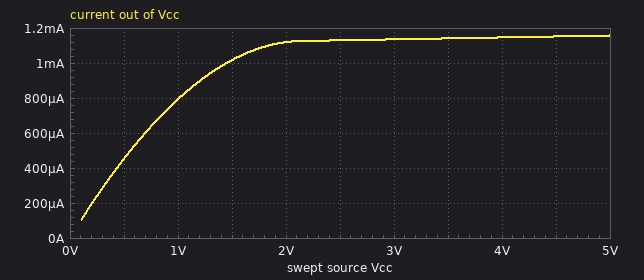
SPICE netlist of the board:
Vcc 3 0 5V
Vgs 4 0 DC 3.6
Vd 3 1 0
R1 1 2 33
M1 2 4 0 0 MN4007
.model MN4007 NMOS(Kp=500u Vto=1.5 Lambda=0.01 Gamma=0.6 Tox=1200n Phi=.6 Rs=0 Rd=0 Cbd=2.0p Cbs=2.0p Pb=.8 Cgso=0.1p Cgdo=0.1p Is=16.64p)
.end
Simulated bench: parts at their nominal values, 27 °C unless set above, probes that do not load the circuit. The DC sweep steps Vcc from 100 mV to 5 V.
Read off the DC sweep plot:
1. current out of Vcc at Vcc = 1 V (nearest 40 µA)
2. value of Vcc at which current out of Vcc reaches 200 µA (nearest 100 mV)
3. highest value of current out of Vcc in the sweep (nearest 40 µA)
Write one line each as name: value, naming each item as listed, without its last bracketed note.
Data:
current out of Vcc at Vcc = 1 V: 800 µA
value of Vcc at which current out of Vcc reaches 200 µA: 200 mV
highest value of current out of Vcc in the sweep: 1.16 mA
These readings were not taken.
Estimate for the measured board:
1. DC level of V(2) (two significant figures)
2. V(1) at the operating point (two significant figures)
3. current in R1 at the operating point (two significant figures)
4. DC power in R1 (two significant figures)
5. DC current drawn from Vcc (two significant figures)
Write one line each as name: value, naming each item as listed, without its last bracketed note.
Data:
DC level of V(2): 5.0 V
V(1) at the operating point: 5.0 V
current in R1 at the operating point: 1.2 mA
DC power in R1: 44 µW
DC current drawn from Vcc: 1.2 mA
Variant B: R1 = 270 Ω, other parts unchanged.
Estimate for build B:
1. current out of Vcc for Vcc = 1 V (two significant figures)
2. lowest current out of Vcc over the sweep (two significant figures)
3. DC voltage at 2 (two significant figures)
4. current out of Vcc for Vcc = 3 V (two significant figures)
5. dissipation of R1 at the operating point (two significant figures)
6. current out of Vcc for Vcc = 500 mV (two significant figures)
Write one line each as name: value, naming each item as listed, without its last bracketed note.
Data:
current out of Vcc for Vcc = 1 V: 690 µA
lowest current out of Vcc over the sweep: 81 µA
DC voltage at 2: 4.7 V
current out of Vcc for Vcc = 3 V: 1.1 mA
dissipation of R1 at the operating point: 360 µW
current out of Vcc for Vcc = 500 mV: 380 µA
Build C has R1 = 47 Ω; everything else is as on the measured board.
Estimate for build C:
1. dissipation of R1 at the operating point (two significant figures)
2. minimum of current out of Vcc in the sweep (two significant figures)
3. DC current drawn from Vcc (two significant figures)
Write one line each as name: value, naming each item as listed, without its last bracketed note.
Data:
dissipation of R1 at the operating point: 63 µW
minimum of current out of Vcc in the sweep: 98 µA
DC current drawn from Vcc: 1.2 mA
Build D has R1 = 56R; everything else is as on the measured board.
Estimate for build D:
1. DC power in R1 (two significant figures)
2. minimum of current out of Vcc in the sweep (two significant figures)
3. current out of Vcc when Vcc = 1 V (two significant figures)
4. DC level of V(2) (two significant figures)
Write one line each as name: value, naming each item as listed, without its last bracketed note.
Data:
DC power in R1: 75 µW
minimum of current out of Vcc in the sweep: 97 µA
current out of Vcc when Vcc = 1 V: 780 µA
DC level of V(2): 4.9 V
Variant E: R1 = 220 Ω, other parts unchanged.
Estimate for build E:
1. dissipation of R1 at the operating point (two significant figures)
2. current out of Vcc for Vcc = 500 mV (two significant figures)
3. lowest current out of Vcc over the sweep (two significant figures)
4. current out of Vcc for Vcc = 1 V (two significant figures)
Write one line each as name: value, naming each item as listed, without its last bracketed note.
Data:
dissipation of R1 at the operating point: 290 µW
current out of Vcc for Vcc = 500 mV: 390 µA
lowest current out of Vcc over the sweep: 84 µA
current out of Vcc for Vcc = 1 V: 710 µA
